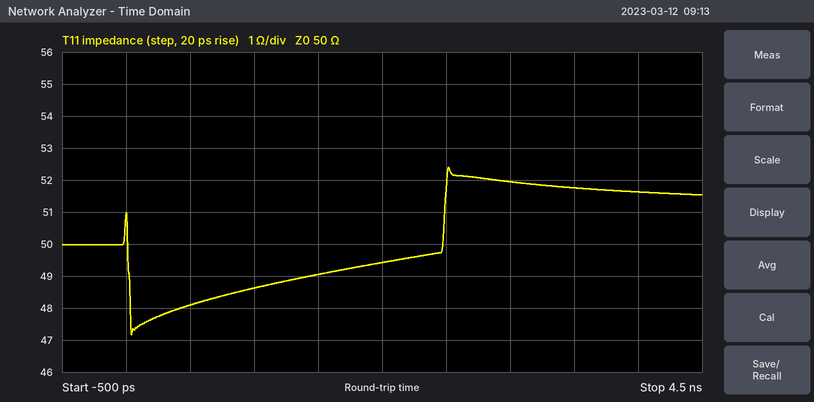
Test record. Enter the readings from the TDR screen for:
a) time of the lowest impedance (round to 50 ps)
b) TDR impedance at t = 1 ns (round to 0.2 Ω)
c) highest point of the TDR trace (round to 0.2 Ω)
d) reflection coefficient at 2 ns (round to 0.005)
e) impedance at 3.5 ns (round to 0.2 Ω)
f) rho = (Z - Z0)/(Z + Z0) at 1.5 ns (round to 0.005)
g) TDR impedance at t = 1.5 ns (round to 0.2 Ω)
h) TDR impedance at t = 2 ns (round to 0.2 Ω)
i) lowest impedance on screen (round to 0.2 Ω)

50 ps
48.6 Ω
52.4 Ω
-0.005
51.8 Ω
-0.010
49.0 Ω
49.4 Ω
47.2 Ω
